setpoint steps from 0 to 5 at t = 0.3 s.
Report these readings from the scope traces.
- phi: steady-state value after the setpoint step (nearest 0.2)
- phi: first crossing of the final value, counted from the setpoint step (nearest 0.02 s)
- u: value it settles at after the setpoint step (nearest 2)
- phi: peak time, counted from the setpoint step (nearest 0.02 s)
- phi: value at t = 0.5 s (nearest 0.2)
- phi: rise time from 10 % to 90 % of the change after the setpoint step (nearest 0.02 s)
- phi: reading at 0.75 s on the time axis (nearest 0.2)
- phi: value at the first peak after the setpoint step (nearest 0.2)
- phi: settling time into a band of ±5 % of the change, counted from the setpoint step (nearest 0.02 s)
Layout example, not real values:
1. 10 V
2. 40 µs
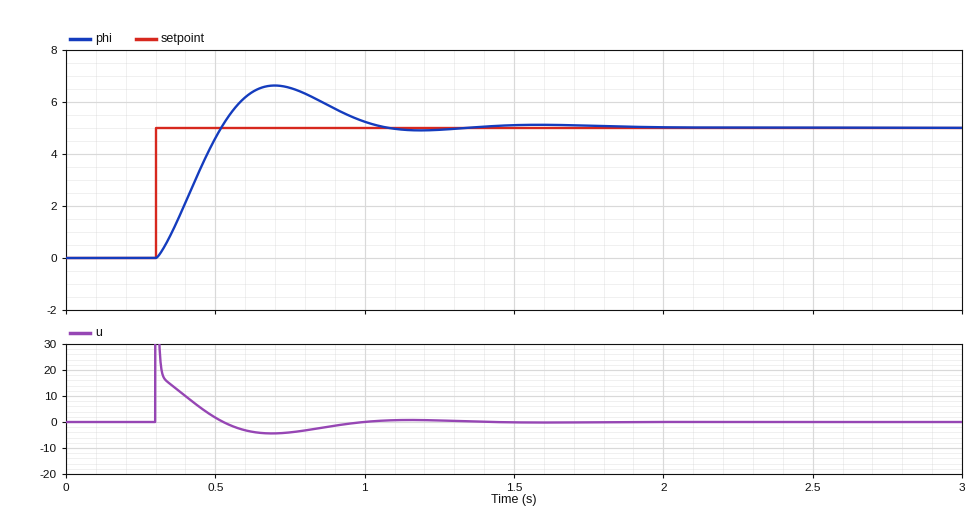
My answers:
1. 5.0
2. 0.22 s
3. 0
4. 0.40 s
5. 4.6
6. 0.16 s
7. 6.6
8. 6.6
9. 0.70 s
